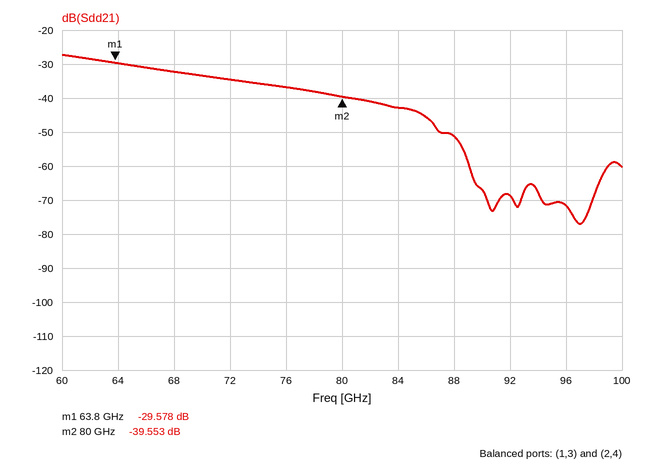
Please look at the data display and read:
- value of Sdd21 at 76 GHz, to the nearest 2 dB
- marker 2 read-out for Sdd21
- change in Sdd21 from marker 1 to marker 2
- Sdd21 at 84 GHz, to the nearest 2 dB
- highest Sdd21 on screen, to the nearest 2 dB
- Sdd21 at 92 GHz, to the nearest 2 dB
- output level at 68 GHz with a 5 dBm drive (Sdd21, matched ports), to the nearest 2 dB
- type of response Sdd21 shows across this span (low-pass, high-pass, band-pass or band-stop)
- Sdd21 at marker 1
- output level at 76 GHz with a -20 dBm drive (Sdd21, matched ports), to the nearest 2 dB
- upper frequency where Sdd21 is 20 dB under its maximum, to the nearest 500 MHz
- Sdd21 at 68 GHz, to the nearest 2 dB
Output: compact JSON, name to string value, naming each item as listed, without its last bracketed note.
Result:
{"value of Sdd21 at 76 GHz, to the nearest 2 dB": "-36 dB", "marker 2 read-out for Sdd21": "-39.553 dB", "change in Sdd21 from marker 1 to marker 2": "-9.975 dB", "Sdd21 at 84 GHz, to the nearest 2 dB": "-42 dB", "highest Sdd21 on screen, to the nearest 2 dB": "-28 dB", "Sdd21 at 92 GHz, to the nearest 2 dB": "-68 dB", "output level at 68 GHz with a 5 dBm drive (Sdd21, matched ports), to the nearest 2 dB": "-28 dBm", "type of response Sdd21 shows across this span": "low-pass", "Sdd21 at marker 1": "-29.578 dB", "output level at 76 GHz with a -20 dBm drive (Sdd21, matched ports), to the nearest 2 dB": "-56 dBm", "upper frequency where Sdd21 is 20 dB under its maximum, to the nearest 500 MHz": "86.5 GHz", "Sdd21 at 68 GHz, to the nearest 2 dB": "-32 dB"}
